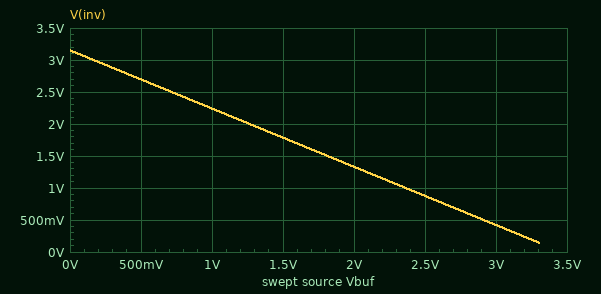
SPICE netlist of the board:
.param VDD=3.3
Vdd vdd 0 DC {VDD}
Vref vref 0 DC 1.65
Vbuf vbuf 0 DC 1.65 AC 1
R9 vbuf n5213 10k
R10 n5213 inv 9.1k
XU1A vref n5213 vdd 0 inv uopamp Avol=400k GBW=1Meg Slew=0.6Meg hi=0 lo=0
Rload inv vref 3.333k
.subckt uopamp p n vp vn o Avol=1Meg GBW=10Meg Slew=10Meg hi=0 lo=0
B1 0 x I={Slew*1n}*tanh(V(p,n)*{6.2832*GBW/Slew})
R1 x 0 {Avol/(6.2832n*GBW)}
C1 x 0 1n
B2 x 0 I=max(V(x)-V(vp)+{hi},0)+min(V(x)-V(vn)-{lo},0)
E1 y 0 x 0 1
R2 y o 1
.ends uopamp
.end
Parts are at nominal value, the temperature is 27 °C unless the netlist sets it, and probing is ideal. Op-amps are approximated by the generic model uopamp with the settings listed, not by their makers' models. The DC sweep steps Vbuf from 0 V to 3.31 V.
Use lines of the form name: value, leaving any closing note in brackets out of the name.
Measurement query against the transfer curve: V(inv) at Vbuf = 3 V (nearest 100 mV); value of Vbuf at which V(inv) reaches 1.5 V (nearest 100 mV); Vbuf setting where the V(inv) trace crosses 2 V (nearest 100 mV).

V(inv) at Vbuf = 3 V: 400 mV
value of Vbuf at which V(inv) reaches 1.5 V: 1.8 V
Vbuf setting where the V(inv) trace crosses 2 V: 1.3 V
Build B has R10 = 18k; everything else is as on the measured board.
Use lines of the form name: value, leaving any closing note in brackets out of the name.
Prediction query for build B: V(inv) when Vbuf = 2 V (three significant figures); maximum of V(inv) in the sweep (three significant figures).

V(inv) when Vbuf = 2 V: 1.02 V
maximum of V(inv) in the sweep: 3.30 V
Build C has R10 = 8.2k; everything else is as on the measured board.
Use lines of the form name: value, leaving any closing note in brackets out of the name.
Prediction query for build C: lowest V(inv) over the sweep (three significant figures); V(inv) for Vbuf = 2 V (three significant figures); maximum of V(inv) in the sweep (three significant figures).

lowest V(inv) over the sweep: 289 mV
V(inv) for Vbuf = 2 V: 1.36 V
maximum of V(inv) in the sweep: 3.00 V
